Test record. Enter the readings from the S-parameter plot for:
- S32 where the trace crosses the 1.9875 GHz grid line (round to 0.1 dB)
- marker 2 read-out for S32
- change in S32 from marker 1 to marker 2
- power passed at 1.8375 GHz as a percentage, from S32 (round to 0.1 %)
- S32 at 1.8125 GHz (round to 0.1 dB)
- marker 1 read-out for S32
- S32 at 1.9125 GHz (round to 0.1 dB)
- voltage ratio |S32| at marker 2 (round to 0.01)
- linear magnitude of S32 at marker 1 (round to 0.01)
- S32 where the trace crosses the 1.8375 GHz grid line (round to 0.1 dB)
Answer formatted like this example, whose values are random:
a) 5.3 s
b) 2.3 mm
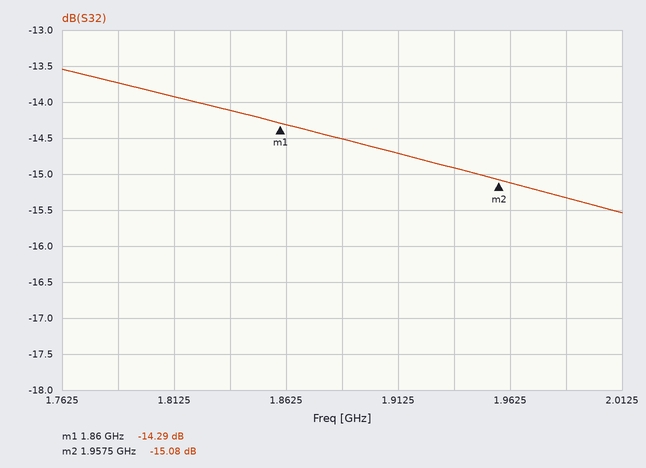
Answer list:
a) -15.3 dB
b) -15.08 dB
c) -0.79 dB
d) 3.9 %
e) -13.9 dB
f) -14.29 dB
g) -14.7 dB
h) 0.18
i) 0.19
j) -14.1 dB
